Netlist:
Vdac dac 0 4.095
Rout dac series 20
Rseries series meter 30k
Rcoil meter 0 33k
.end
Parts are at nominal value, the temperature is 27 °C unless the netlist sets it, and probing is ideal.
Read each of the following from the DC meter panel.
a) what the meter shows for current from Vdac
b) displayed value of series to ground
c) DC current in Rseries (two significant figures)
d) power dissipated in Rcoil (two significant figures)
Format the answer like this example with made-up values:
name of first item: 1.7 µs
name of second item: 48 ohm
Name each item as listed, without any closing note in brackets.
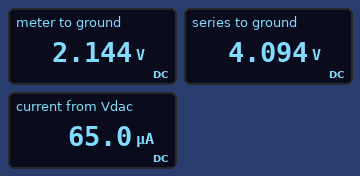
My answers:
what the meter shows for current from Vdac: 65.0 µA
displayed value of series to ground: 4.094 V
DC current in Rseries: 65 µA
power dissipated in Rcoil: 140 µW
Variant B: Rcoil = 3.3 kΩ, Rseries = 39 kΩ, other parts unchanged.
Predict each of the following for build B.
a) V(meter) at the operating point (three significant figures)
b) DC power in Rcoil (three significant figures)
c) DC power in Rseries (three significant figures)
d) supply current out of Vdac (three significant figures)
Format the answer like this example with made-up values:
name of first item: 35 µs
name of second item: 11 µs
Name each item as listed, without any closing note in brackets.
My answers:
V(meter) at the operating point: 319 mV
DC power in Rcoil: 30.9 µW
DC power in Rseries: 365 µW
supply current out of Vdac: 96.8 µA
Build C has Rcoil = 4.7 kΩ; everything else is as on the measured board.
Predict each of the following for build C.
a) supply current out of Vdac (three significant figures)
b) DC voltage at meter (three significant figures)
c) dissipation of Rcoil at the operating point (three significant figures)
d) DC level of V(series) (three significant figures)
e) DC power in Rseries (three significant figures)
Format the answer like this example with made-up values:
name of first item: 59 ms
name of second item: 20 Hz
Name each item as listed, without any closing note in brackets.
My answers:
supply current out of Vdac: 118 µA
DC voltage at meter: 554 mV
dissipation of Rcoil at the operating point: 65.4 µW
DC level of V(series): 4.09 V
DC power in Rseries: 417 µW
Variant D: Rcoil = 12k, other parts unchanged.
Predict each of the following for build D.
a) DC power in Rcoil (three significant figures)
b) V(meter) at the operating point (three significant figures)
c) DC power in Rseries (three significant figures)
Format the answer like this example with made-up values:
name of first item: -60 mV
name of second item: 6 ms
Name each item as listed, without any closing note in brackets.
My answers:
DC power in Rcoil: 114 µW
V(meter) at the operating point: 1.17 V
DC power in Rseries: 285 µW
